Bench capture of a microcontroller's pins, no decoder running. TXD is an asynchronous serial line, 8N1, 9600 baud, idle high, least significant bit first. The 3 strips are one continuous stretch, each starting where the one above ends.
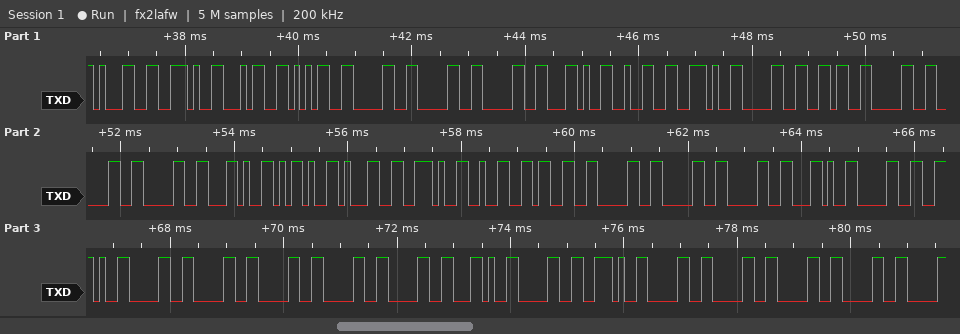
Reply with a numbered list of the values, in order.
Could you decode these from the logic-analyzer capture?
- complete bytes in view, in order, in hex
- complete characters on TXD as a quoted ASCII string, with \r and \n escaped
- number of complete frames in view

1. 31 2E 34 35 30 30 30 2C 32 2E 30 36 30 30 30 2C 2D 31 2E 32 33 30 30 30 2C 30 2E 30 30 30 30 30 2C 30 2E 30 30 30 30
2. "1.45000,2.06000,-1.23000,0.00000,0.0000"
3. 39
